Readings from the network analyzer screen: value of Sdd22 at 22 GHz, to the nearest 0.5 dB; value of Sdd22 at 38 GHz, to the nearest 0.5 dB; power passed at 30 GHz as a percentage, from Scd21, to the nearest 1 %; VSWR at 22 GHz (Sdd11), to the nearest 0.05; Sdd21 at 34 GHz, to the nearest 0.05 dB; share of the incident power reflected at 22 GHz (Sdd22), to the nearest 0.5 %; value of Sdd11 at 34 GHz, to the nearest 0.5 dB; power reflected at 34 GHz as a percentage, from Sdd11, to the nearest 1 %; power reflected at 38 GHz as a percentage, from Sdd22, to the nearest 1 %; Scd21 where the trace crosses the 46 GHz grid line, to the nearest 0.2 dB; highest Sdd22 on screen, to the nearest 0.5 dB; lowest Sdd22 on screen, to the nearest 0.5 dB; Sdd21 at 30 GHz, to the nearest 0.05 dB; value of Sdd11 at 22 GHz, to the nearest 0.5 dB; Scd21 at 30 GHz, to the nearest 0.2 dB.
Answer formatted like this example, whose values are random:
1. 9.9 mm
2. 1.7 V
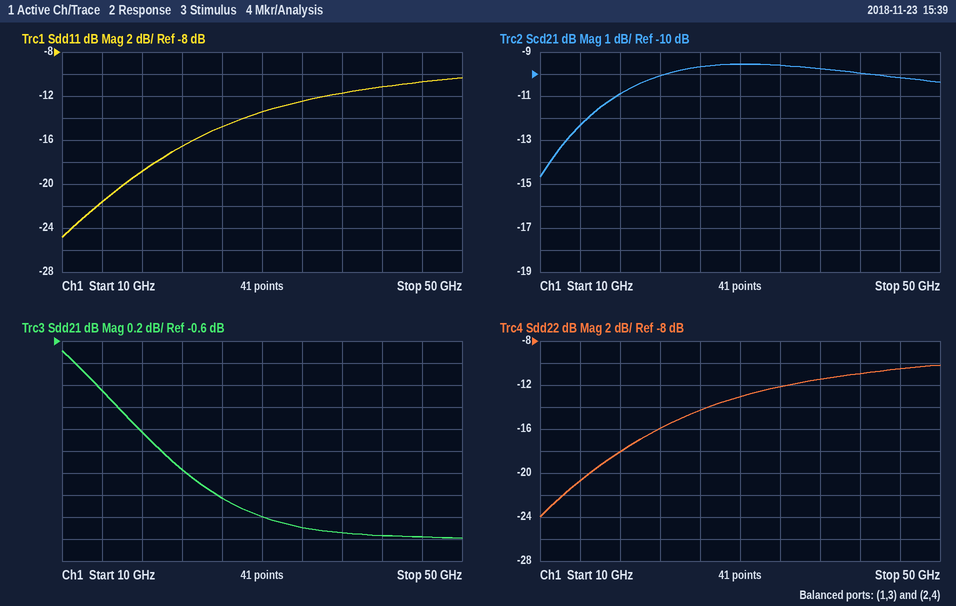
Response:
1. -16.0 dB
2. -11.5 dB
3. 11 %
4. 1.35
5. -2.30 dB
6. 2.5 %
7. -12.5 dB
8. 6 %
9. 7 %
10. -10.2 dB
11. -10.0 dB
12. -24.0 dB
13. -2.20 dB
14. -16.5 dB
15. -9.6 dB
